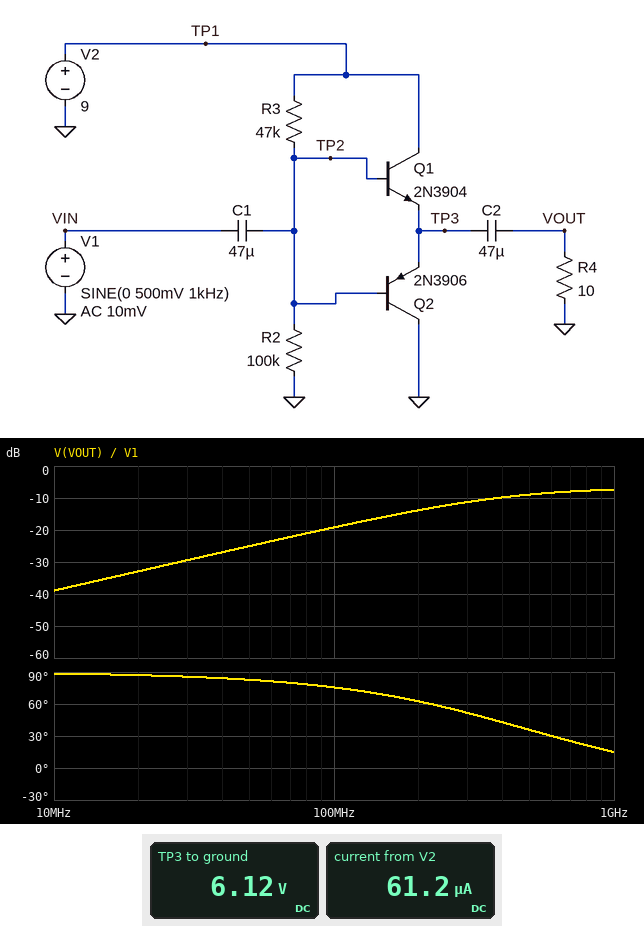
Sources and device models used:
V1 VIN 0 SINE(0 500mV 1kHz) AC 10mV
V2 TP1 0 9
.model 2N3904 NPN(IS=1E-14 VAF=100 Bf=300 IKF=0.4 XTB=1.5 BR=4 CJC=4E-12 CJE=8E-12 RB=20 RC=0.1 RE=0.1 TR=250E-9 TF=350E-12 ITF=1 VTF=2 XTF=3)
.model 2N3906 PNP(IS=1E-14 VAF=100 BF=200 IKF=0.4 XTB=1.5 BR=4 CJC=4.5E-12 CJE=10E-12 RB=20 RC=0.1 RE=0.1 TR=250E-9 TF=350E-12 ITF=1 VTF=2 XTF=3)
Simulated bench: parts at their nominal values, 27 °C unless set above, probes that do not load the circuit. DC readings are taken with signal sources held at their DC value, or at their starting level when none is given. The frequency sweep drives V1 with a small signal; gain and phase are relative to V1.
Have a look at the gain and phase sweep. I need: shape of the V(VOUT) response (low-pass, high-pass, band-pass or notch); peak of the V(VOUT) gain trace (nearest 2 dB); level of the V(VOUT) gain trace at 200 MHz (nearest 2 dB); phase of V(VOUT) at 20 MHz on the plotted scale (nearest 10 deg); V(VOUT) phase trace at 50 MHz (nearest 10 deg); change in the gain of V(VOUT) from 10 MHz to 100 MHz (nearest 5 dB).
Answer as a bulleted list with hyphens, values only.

- high-pass
- -8 dB
- -14 dB
- 90 deg
- 80 deg
- 20 dB
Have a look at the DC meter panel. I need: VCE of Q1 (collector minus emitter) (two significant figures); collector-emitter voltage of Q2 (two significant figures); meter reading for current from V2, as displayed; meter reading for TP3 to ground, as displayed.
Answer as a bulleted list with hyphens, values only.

- 2.9 V
- -6.1 V
- 61.2 µA
- 6.12 V
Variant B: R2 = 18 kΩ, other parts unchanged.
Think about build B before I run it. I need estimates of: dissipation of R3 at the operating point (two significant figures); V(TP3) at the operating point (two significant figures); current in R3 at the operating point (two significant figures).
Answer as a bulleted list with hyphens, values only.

- 900 µW
- 2.5 V
- 140 µA
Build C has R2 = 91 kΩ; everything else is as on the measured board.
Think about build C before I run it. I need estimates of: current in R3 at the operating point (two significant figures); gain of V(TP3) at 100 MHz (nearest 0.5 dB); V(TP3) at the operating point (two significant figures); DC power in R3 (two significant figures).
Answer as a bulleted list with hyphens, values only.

- 65 µA
- -19.0 dB
- 5.9 V
- 200 µW
